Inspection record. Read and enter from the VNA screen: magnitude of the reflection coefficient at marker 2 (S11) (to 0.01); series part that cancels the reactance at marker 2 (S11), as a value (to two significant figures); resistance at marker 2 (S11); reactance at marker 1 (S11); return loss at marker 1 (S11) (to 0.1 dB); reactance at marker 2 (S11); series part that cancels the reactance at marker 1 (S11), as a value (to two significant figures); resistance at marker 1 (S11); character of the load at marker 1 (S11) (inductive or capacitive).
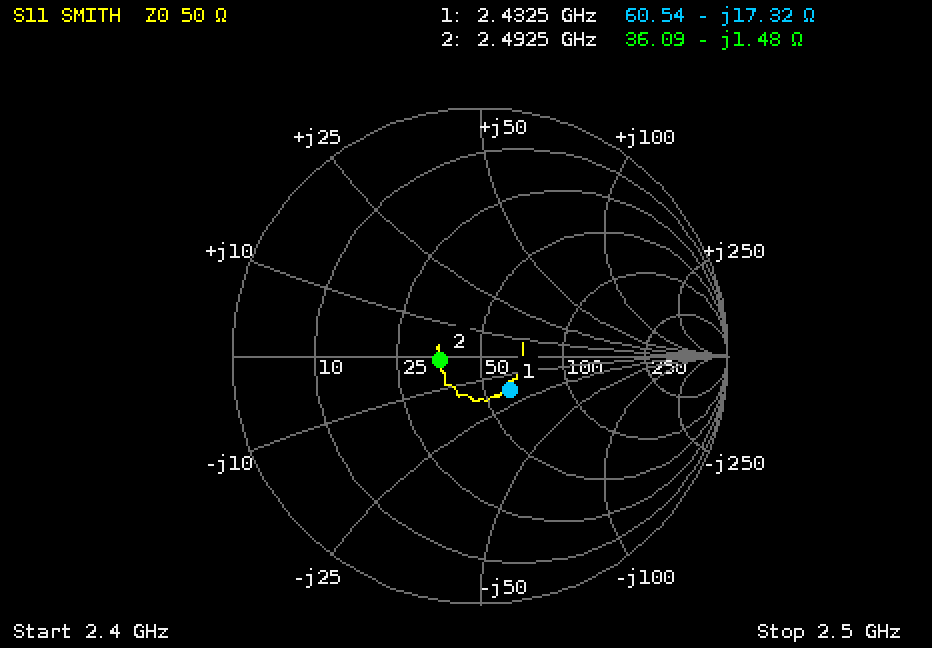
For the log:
0.16
95 pH
36.09 Ω
-17.32 Ω
14.8 dB
-1.48 Ω
1.1 nH
60.54 Ω
capacitive
